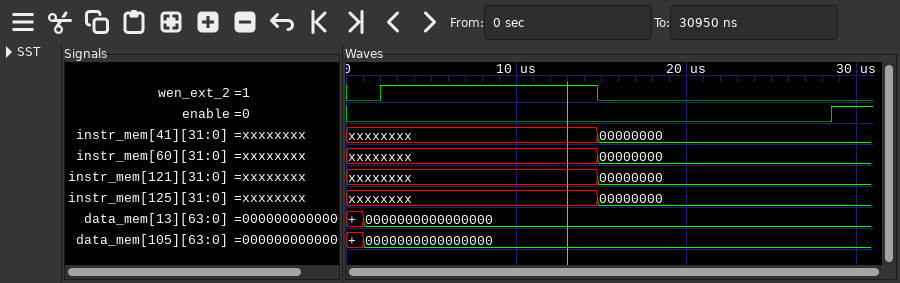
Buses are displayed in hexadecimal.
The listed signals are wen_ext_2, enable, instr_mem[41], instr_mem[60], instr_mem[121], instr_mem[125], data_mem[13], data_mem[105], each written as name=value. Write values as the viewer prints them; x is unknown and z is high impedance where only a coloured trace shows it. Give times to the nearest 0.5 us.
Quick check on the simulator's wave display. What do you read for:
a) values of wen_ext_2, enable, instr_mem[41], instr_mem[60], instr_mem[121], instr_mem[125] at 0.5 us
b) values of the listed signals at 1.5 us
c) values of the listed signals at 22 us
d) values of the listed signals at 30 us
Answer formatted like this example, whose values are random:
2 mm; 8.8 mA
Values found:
wen_ext_2=0, enable=0, instr_mem[41]=xxxxxxxx, instr_mem[60]=xxxxxxxx, instr_mem[121]=xxxxxxxx, instr_mem[125]=xxxxxxxx; wen_ext_2=0, enable=0, instr_mem[41]=xxxxxxxx, instr_mem[60]=xxxxxxxx, instr_mem[121]=xxxxxxxx, instr_mem[125]=xxxxxxxx, data_mem[13]=0000000000000000, data_mem[105]=0000000000000000; wen_ext_2=0, enable=0, instr_mem[41]=00000000, instr_mem[60]=00000000, instr_mem[121]=00000000, instr_mem[125]=00000000, data_mem[13]=0000000000000000, data_mem[105]=0000000000000000; wen_ext_2=0, enable=1, instr_mem[41]=00000000, instr_mem[60]=00000000, instr_mem[121]=00000000, instr_mem[125]=00000000, data_mem[13]=0000000000000000, data_mem[105]=0000000000000000
